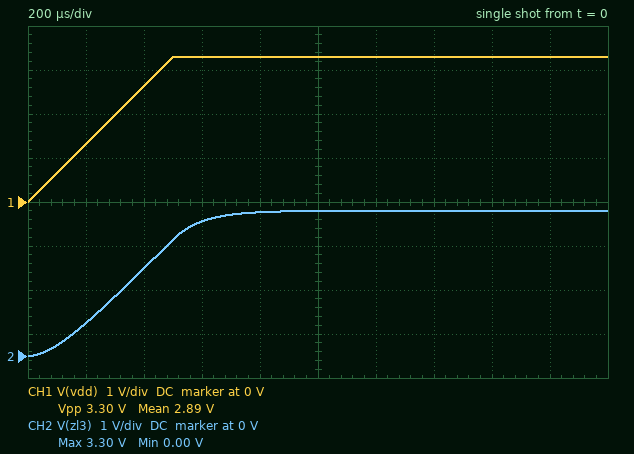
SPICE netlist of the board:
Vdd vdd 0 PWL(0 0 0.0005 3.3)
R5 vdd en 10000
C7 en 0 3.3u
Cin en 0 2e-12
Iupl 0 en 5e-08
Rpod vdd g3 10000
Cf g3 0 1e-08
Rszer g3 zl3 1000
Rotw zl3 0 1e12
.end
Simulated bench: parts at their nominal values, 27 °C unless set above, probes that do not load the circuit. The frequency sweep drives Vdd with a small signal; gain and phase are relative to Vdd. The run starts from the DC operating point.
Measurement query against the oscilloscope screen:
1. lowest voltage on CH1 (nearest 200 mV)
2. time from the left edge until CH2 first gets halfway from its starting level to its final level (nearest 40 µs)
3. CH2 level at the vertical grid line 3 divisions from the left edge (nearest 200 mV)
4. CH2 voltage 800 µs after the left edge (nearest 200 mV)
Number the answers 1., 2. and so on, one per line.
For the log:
1. 0 V
2. 360 µs
3. 3.0 V
4. 3.2 V
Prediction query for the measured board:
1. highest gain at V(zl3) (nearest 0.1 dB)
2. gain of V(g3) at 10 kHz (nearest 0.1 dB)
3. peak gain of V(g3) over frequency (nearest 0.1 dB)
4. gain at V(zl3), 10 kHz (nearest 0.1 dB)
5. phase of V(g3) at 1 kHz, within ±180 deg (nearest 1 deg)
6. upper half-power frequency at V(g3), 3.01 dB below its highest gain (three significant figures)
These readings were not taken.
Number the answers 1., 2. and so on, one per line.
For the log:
1. 0 dB
2. -16.1 dB
3. 0 dB
4. -16.1 dB
5. -32 deg
6. 1.59 kHz
